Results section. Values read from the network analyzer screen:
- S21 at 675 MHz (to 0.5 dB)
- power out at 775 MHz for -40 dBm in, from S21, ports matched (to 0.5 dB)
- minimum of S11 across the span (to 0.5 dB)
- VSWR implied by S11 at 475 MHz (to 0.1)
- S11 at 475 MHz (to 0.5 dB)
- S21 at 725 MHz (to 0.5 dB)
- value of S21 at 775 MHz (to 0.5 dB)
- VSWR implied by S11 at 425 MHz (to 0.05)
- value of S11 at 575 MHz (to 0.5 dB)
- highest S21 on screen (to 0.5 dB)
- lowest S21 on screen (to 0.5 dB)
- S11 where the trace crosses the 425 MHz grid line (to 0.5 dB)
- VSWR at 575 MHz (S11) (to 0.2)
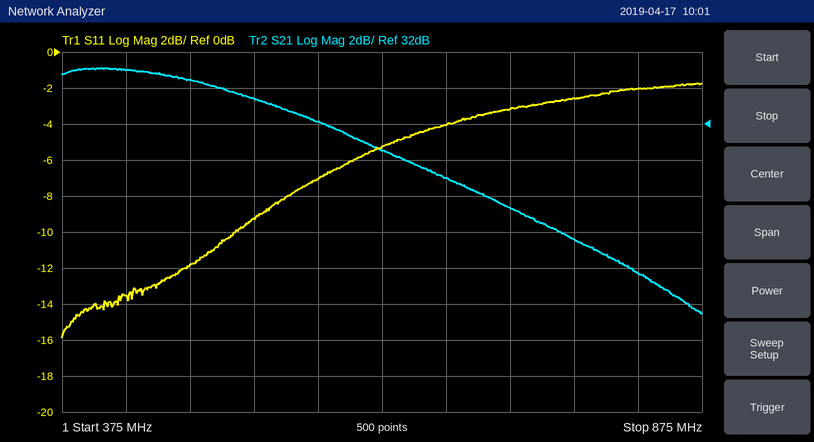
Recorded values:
29.0 dB
-14.5 dBm
-16.0 dB
1.7
-12.0 dB
27.5 dB
25.5 dB
1.55
-7.0 dB
35.0 dB
21.5 dB
-13.5 dB
2.6
